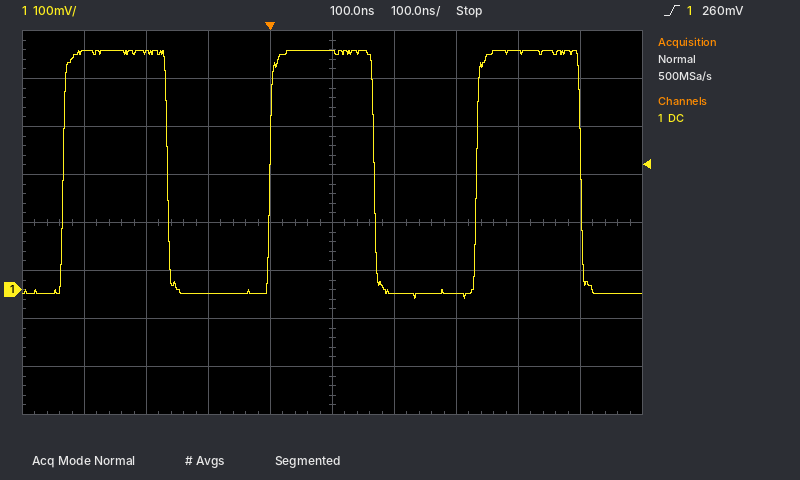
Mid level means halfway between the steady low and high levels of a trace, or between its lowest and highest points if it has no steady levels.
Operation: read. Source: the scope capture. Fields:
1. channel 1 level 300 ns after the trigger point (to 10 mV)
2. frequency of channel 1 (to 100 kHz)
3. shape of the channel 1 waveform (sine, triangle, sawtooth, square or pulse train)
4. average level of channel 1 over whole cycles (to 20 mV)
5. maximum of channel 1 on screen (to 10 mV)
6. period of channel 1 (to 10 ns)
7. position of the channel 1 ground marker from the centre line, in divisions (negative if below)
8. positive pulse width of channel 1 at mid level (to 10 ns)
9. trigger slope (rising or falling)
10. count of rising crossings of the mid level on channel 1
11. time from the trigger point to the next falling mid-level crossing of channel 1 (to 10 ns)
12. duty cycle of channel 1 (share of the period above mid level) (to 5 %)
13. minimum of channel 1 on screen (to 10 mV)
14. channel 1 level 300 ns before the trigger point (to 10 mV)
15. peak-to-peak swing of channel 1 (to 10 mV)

-10 mV
3.0 MHz
square
240 mV
500 mV
330 ns
-1.4 div
170 ns
rising
3
170 ns
50 %
-20 mV
500 mV
520 mV
